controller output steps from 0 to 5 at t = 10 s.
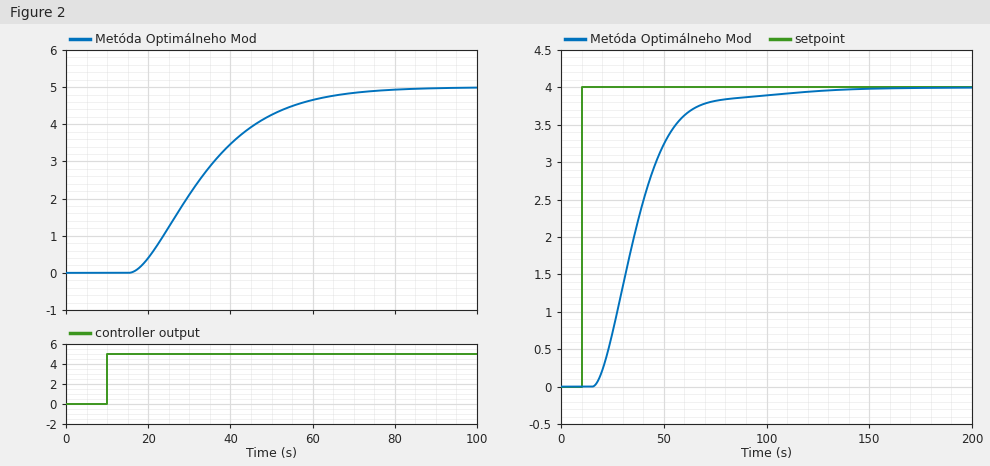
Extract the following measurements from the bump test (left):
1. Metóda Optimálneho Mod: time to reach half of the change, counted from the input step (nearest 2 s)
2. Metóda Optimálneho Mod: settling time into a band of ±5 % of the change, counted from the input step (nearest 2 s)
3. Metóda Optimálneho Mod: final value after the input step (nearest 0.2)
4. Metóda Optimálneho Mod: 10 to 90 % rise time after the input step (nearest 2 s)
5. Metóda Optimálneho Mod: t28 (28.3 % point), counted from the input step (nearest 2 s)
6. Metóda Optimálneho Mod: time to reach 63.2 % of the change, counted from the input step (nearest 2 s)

22 s
54 s
5.0
34 s
16 s
28 s
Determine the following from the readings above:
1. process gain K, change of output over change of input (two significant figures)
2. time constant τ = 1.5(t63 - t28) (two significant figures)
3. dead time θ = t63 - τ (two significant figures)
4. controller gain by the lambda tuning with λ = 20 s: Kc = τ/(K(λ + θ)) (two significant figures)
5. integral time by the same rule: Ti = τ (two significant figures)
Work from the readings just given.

1.0
18 s
10 s
0.60
18 s
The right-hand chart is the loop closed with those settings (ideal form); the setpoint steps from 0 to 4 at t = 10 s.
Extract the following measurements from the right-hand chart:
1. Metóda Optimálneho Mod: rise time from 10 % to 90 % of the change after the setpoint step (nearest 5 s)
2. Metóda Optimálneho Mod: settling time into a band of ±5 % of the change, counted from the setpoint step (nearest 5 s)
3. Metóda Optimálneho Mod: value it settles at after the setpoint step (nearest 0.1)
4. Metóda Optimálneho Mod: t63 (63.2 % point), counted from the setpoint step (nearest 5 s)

35 s
60 s
4.0
30 s
